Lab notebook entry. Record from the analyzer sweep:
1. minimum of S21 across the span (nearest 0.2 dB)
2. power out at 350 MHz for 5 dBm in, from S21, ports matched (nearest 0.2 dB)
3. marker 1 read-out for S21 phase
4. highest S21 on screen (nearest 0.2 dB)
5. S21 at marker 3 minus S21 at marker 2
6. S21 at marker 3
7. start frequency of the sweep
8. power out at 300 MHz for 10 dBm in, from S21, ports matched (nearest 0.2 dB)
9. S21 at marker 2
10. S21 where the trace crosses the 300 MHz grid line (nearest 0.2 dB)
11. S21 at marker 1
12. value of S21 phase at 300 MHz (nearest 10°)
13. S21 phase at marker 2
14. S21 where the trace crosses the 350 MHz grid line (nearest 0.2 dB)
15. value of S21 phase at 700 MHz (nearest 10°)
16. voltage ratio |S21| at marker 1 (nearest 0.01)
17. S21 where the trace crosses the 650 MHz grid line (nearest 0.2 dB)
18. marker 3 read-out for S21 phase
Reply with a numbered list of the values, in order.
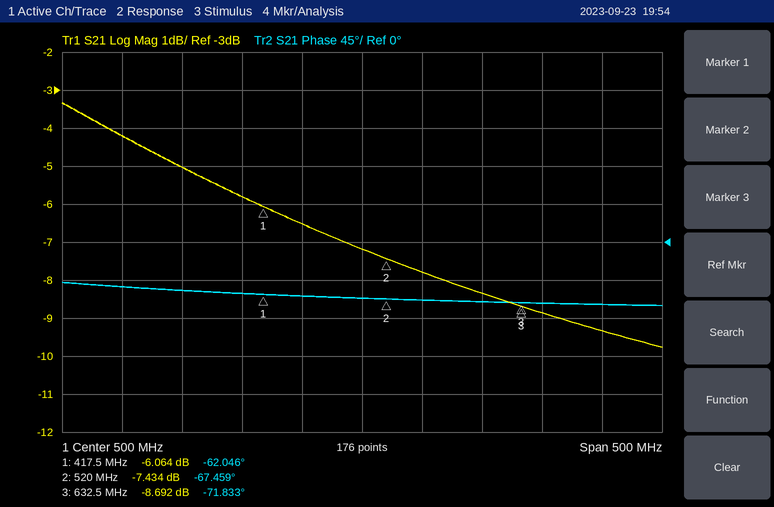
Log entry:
1. -9.8 dB
2. 0.0 dBm
3. -62.046°
4. -3.4 dB
5. -1.258 dB
6. -8.692 dB
7. 250 MHz
8. 5.8 dBm
9. -7.434 dB
10. -4.2 dB
11. -6.064 dB
12. -50°
13. -67.459°
14. -5.0 dB
15. -70°
16. 0.50
17. -8.8 dB
18. -71.833°
